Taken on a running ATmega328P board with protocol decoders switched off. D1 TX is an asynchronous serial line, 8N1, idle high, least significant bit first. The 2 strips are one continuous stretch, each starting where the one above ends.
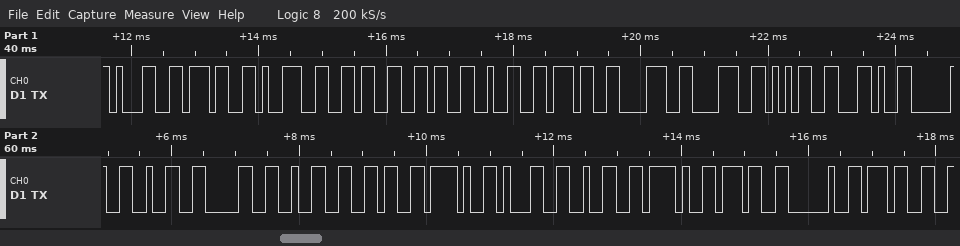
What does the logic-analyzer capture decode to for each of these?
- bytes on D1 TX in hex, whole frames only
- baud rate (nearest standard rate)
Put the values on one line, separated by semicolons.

0x31 0x37 0x39 0x36 0x36 0x32 0x37 0x38 0x38 0x35 0x2C 0x20 0x32 0x30 0x32 0x36 0x2F 0x31 0x32 0x2F 0x37 0x20 0x37; 9600 baud
